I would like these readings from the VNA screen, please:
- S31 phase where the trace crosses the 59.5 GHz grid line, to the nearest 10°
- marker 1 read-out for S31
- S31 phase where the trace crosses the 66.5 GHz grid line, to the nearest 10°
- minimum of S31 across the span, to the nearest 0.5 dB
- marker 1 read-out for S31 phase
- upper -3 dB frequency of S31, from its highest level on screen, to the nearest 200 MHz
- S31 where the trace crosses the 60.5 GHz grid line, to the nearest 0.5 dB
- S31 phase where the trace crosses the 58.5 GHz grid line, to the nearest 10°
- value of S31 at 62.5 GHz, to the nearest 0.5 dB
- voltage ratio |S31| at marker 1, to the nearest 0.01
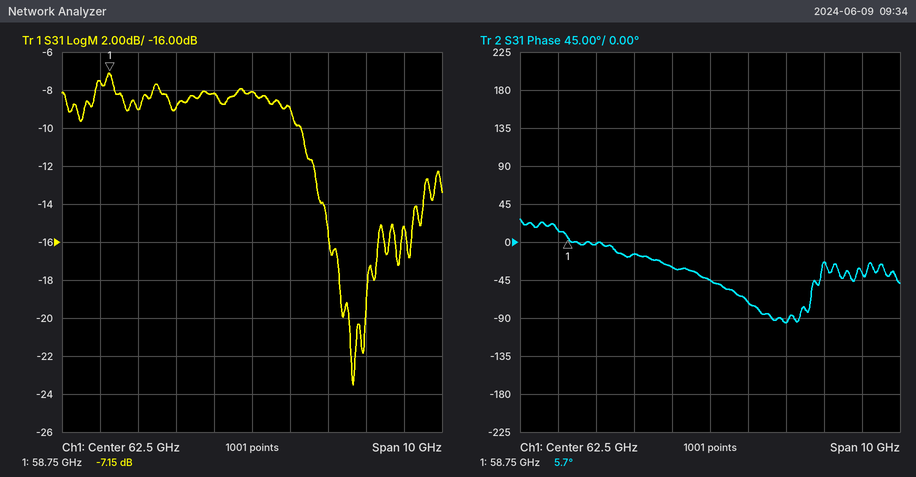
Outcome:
0°
-7.15 dB
-40°
-23.5 dB
5.7°
63.8 GHz
-9.0 dB
10°
-8.0 dB
0.44
